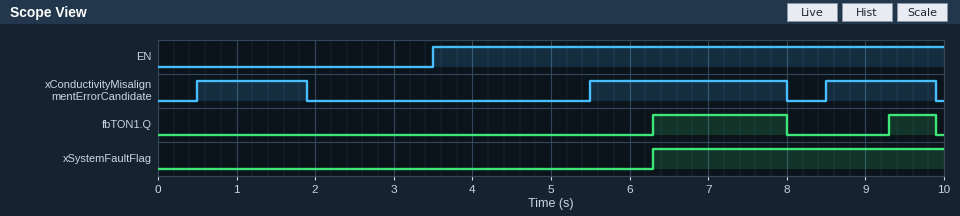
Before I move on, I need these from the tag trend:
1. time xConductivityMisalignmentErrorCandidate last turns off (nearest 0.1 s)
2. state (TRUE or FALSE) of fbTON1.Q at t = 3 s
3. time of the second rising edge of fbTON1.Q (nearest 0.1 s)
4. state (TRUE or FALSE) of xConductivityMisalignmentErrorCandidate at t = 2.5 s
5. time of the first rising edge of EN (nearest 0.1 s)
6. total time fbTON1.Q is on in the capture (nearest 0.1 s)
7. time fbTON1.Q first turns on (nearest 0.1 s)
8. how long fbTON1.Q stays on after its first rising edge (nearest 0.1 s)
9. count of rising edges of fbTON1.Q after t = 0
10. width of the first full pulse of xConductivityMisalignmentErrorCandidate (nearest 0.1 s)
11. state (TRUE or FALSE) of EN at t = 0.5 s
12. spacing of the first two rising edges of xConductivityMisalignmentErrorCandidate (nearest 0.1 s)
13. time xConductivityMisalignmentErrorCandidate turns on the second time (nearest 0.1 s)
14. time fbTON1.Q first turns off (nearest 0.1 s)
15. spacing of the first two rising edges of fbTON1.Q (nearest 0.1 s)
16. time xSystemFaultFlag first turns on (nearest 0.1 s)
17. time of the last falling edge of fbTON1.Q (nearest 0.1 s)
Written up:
9.9 s
FALSE
9.3 s
FALSE
3.5 s
2.3 s
6.3 s
1.7 s
2
1.4 s
FALSE
5.0 s
5.5 s
8.0 s
3.0 s
6.3 s
9.9 s
